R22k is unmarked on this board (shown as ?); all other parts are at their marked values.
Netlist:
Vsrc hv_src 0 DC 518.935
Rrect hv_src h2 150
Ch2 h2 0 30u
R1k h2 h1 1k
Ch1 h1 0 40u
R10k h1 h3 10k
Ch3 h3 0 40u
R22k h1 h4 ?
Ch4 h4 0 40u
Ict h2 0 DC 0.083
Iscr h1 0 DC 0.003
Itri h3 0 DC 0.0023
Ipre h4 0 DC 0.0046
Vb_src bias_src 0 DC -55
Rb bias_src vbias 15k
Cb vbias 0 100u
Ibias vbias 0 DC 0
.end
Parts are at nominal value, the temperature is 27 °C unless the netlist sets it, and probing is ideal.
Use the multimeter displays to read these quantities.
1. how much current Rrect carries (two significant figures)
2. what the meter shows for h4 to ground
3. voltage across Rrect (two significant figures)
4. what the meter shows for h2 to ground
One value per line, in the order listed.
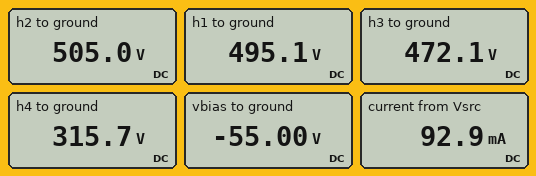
93 mA
315.7 V
14 V
505.0 V
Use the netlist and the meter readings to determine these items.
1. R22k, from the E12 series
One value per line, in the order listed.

39 kΩ
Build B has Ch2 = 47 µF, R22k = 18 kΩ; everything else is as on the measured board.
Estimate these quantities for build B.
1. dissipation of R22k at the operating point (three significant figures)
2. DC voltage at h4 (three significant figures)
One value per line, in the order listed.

381 mW
412 V
